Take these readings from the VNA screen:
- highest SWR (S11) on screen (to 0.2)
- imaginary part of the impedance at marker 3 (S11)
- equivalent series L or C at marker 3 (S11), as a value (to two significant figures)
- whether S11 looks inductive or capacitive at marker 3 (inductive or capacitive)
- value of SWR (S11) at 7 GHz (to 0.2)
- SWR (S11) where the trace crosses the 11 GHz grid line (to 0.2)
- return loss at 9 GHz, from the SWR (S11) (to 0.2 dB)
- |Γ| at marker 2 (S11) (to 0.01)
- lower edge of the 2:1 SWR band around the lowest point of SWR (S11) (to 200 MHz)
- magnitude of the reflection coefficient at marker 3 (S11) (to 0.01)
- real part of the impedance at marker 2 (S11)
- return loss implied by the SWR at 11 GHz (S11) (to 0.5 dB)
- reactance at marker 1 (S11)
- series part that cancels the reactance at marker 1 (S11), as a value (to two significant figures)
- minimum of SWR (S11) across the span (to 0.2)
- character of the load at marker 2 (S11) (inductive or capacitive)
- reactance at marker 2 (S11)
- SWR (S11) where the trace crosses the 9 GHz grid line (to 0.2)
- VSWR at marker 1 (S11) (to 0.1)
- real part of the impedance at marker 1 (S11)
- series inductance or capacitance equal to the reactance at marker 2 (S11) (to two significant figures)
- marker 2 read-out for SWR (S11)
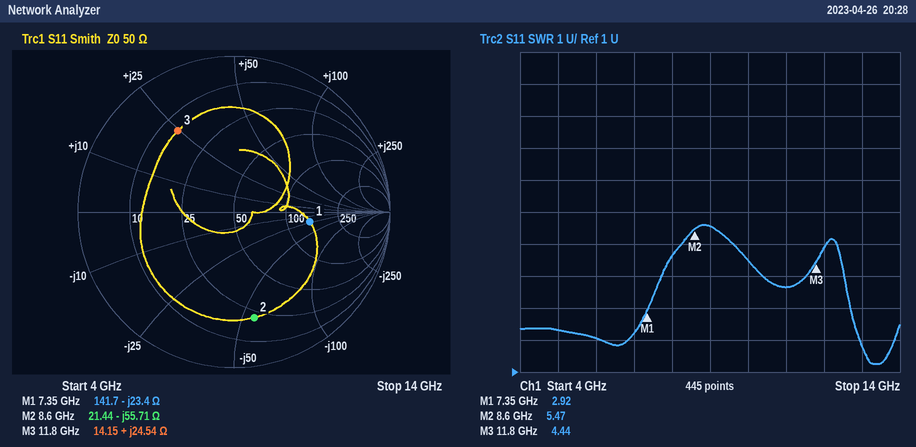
5.6
+24.54 Ω
330 pH
inductive
2.2
3.6
3.2 dB
0.69
13.0 GHz
0.63
21.44 Ω
5.0 dB
-23.4 Ω
510 pH
1.2
capacitive
-55.71 Ω
5.6
2.9
141.7 Ω
330 fF
5.47
